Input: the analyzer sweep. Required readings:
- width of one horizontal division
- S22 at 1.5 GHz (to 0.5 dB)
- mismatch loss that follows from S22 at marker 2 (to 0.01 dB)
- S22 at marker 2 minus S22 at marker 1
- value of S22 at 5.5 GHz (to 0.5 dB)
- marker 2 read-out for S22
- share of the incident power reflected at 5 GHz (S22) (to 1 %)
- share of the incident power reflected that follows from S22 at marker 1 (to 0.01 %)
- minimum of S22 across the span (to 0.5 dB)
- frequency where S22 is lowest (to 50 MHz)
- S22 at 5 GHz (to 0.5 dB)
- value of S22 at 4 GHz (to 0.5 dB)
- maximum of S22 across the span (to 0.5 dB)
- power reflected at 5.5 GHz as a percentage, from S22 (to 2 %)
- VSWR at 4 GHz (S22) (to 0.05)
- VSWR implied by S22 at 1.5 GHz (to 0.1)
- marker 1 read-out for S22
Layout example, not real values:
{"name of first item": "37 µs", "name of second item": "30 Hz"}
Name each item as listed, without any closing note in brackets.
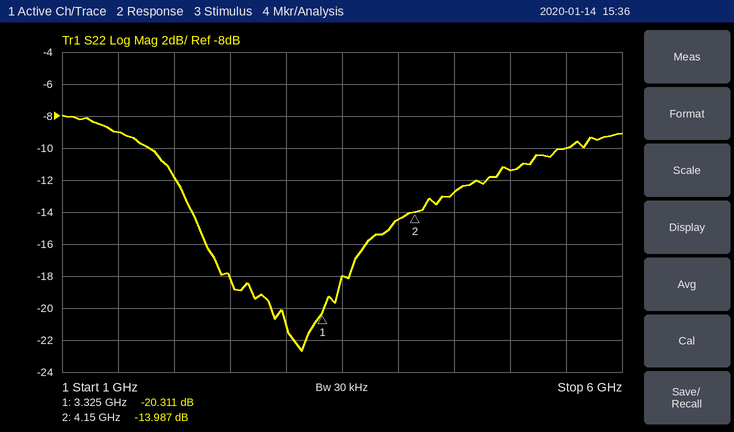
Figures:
{"width of one horizontal division": "500 MHz", "S22 at 1.5 GHz": "-9.0 dB", "mismatch loss that follows from S22 at marker 2": "0.18 dB", "S22 at marker 2 minus S22 at marker 1": "6.324 dB", "value of S22 at 5.5 GHz": "-10.0 dB", "marker 2 read-out for S22": "-13.987 dB", "share of the incident power reflected at 5 GHz (S22)": "7 %", "share of the incident power reflected that follows from S22 at marker 1": "0.93 %", "minimum of S22 across the span": "-22.5 dB", "frequency where S22 is lowest": "3.15 GHz", "S22 at 5 GHz": "-11.5 dB", "value of S22 at 4 GHz": "-14.5 dB", "maximum of S22 across the span": "-8.0 dB", "power reflected at 5.5 GHz as a percentage, from S22": "10 %", "VSWR at 4 GHz (S22)": "1.45", "VSWR implied by S22 at 1.5 GHz": "2.1", "marker 1 read-out for S22": "-20.311 dB"}
